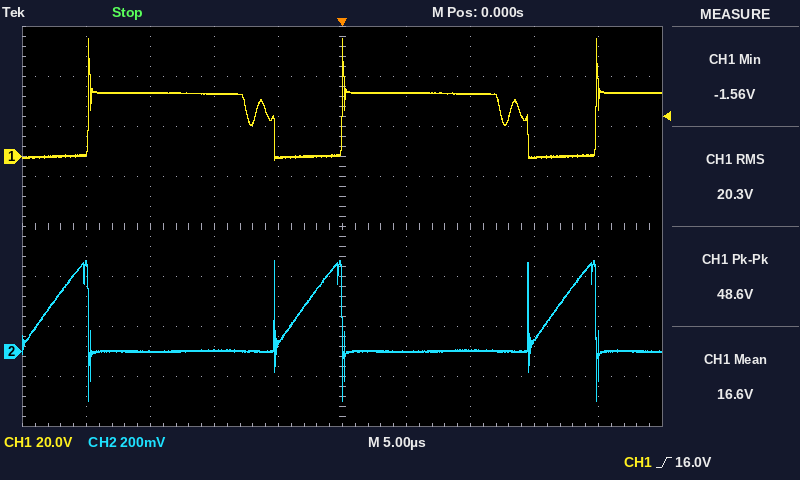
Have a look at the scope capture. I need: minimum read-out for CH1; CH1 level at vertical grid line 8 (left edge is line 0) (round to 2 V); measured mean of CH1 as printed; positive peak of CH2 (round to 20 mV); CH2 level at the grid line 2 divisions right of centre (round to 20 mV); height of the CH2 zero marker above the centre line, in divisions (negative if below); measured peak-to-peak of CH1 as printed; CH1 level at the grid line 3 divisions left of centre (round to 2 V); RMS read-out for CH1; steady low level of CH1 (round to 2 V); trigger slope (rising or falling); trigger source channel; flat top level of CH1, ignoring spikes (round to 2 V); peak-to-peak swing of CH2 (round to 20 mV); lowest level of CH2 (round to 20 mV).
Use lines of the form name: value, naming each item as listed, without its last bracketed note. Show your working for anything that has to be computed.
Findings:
minimum read-out for CH1: -1.56 V
CH1 level at vertical grid line 8 (left edge is line 0): 0 V
measured mean of CH1 as printed: 16.6 V
positive peak of CH2: 360 mV
CH2 level at the grid line 2 divisions right of centre: 0 mV
height of the CH2 zero marker above the centre line, in divisions: -2.5 div
measured peak-to-peak of CH1 as printed: 48.6 V
CH1 level at the grid line 3 divisions left of centre: 26 V
RMS read-out for CH1: 20.3 V
steady low level of CH1: 0 V
trigger slope: rising
trigger source channel: CH1
flat top level of CH1, ignoring spikes: 26 V
peak-to-peak swing of CH2: 360 mV − (-200 mV) = 560 mV
lowest level of CH2: -200 mV
